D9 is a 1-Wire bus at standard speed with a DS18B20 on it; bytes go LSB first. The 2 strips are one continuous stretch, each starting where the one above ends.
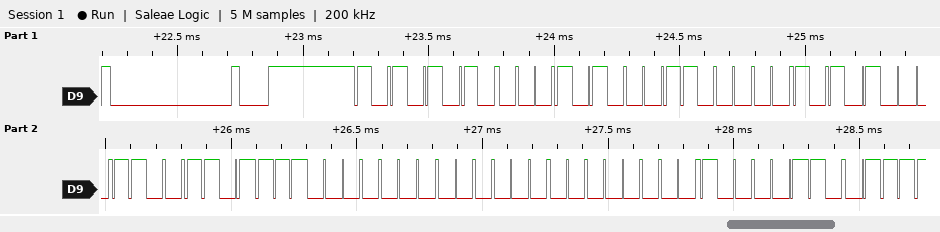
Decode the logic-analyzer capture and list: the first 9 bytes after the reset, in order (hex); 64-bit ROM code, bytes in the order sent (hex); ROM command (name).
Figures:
55 28 06 15 B3 07 00 00 61
28 06 15 B3 07 00 00 61
Match ROM
